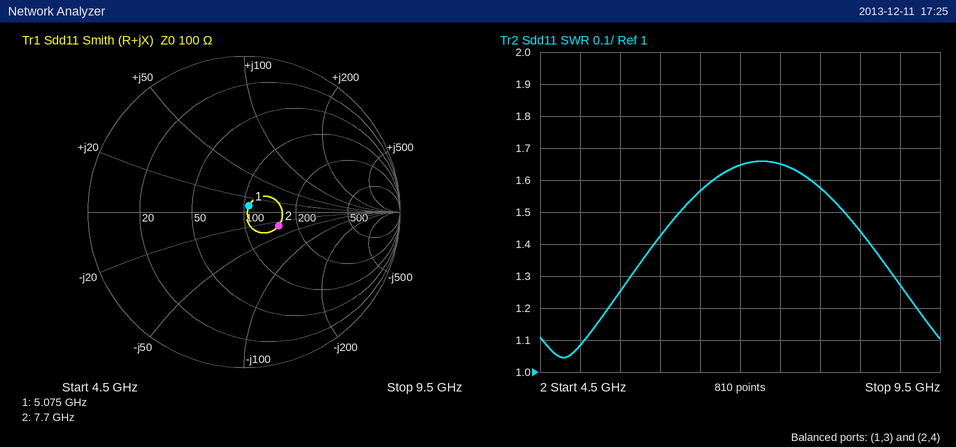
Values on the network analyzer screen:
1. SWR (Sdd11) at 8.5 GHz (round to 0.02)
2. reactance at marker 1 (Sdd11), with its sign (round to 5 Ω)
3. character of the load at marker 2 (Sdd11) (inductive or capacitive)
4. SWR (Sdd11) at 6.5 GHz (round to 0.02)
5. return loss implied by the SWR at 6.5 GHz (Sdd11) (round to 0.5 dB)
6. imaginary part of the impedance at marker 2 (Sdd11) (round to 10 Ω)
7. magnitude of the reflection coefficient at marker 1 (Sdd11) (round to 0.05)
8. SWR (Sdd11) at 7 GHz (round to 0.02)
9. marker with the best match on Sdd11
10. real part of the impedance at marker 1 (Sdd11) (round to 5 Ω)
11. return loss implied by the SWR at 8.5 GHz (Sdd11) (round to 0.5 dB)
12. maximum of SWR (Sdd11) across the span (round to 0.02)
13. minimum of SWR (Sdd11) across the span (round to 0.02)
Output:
1.44
+10 Ω
capacitive
1.56
13.0 dB
-30 Ω
0.05
1.64
marker 1
105 Ω
15.0 dB
1.66
1.04
